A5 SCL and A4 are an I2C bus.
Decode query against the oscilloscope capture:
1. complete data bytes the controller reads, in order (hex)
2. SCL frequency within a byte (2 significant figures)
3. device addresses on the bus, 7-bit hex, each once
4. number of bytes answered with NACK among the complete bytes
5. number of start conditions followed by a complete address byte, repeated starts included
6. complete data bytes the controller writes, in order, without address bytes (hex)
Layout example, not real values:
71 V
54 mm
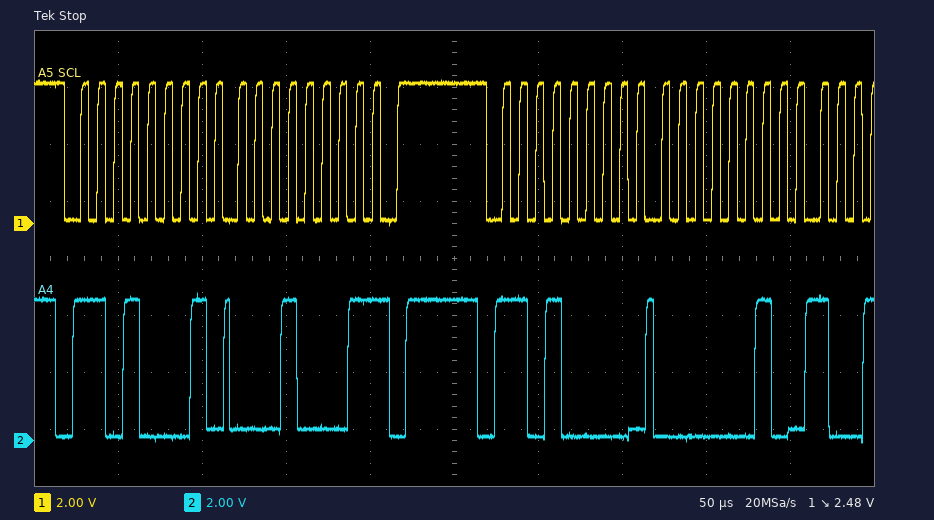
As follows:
11
100 kHz
0x68
1
2
02
